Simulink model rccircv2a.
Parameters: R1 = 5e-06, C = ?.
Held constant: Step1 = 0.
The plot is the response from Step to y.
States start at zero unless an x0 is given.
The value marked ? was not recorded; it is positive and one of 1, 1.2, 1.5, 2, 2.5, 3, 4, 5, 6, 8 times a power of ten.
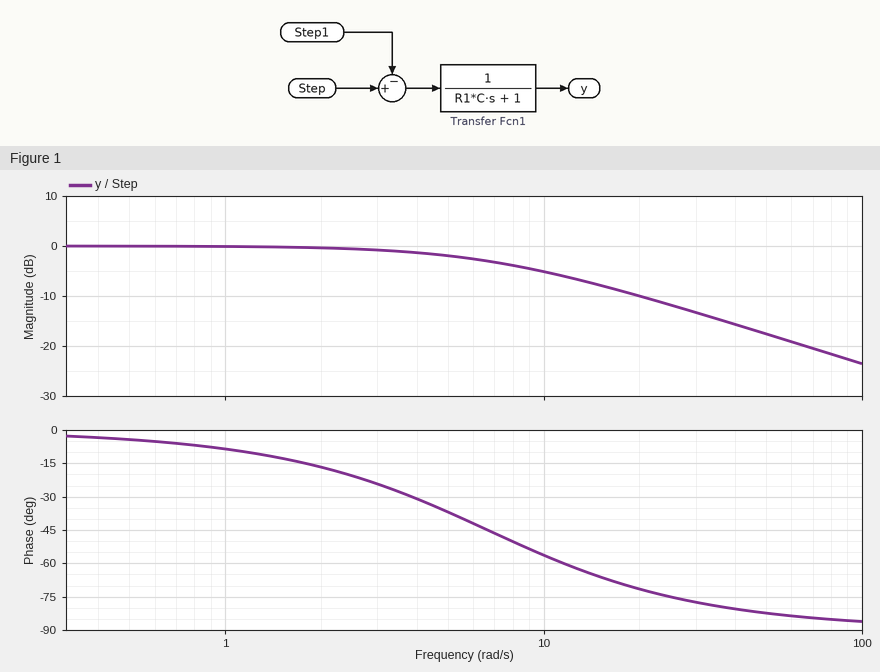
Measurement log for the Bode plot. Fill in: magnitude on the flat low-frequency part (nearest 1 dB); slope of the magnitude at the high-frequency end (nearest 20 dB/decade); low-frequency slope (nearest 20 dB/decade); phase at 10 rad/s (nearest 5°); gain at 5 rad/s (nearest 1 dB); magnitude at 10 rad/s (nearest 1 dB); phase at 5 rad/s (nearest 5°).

0 dB
-20 dB/decade
0 dB/decade
-55°
-2 dB
-5 dB
-35°
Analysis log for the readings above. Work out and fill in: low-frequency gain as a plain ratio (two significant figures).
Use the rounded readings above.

1.0
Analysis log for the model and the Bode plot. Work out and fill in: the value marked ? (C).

30000
